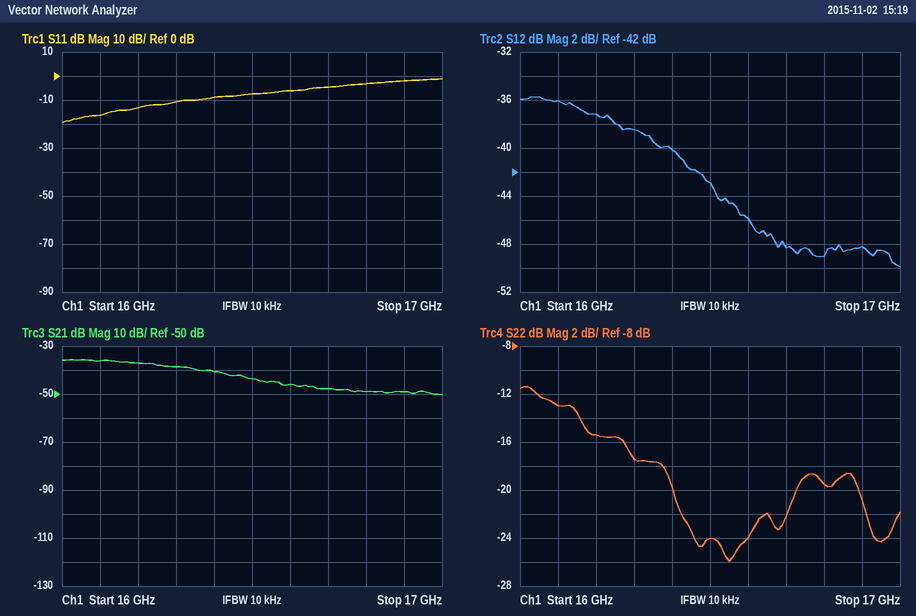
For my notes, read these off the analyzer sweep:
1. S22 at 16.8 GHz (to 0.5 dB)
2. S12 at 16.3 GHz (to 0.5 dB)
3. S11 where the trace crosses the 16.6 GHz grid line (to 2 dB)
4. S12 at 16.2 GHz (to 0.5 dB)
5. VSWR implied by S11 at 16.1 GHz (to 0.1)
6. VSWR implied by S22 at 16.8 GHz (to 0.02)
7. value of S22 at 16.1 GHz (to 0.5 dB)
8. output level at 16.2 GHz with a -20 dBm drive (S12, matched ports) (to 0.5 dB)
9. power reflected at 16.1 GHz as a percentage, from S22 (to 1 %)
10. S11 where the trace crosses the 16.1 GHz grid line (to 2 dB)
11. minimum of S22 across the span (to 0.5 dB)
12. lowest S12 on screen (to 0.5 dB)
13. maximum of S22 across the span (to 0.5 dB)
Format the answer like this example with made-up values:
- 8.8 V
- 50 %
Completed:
- -19.5 dB
- -38.5 dB
- -6 dB
- -37.0 dB
- 1.4
- 1.24
- -13.0 dB
- -57.0 dBm
- 5 %
- -16 dB
- -26.0 dB
- -50.0 dB
- -11.5 dB
